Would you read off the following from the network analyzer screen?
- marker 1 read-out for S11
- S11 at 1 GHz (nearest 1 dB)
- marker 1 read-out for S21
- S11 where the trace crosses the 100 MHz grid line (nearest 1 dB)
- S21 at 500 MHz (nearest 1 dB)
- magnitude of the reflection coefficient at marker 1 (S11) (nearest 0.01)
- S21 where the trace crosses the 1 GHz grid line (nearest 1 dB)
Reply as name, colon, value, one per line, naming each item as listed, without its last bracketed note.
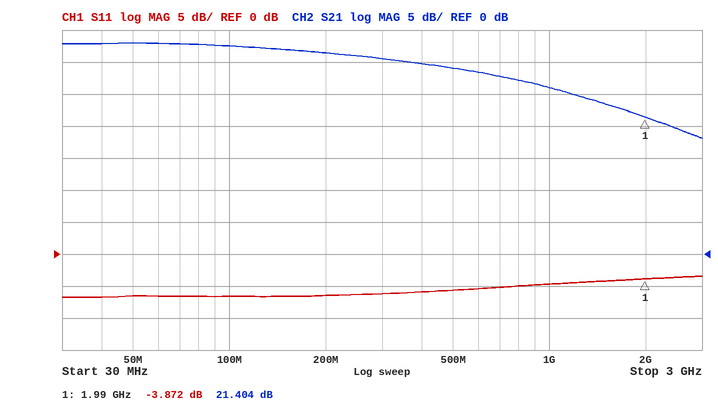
marker 1 read-out for S11: -3.872 dB
S11 at 1 GHz: -5 dB
marker 1 read-out for S21: 21.404 dB
S11 where the trace crosses the 100 MHz grid line: -7 dB
S21 at 500 MHz: 29 dB
magnitude of the reflection coefficient at marker 1 (S11): 0.64
S21 where the trace crosses the 1 GHz grid line: 26 dB
